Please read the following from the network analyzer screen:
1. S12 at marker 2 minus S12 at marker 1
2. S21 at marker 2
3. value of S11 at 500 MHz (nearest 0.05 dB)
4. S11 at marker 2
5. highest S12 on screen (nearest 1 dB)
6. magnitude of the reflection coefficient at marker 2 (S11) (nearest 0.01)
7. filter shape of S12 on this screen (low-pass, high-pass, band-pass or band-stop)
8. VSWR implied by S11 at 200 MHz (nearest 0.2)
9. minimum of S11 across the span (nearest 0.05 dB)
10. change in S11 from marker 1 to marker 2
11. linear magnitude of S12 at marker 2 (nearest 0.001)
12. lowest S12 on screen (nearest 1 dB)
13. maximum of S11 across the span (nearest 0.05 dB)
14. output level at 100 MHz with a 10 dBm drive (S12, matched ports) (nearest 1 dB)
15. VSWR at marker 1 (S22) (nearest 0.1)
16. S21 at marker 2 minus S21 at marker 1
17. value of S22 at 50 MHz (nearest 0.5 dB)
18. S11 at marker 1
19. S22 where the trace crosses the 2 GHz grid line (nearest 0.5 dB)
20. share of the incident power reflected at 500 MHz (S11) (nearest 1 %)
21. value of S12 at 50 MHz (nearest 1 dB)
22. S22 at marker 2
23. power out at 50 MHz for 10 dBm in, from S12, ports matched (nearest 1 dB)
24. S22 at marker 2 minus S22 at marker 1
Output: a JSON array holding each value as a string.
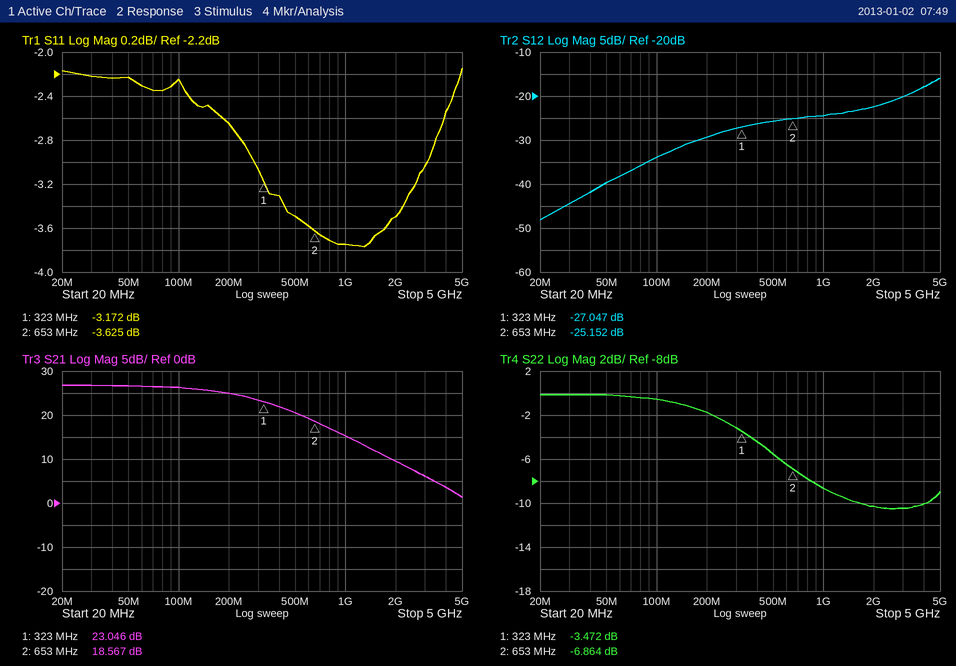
["1.895 dB", "18.567 dB", "-3.50 dB", "-3.625 dB", "-16 dB", "0.66", "high-pass", "6.6", "-3.75 dB", "-0.453 dB", "0.055", "-48 dB", "-2.15 dB", "-24 dBm", "5.1", "-4.479 dB", "0.0 dB", "-3.172 dB", "-10.5 dB", "45 %", "-40 dB", "-6.864 dB", "-30 dBm", "-3.392 dB"]
